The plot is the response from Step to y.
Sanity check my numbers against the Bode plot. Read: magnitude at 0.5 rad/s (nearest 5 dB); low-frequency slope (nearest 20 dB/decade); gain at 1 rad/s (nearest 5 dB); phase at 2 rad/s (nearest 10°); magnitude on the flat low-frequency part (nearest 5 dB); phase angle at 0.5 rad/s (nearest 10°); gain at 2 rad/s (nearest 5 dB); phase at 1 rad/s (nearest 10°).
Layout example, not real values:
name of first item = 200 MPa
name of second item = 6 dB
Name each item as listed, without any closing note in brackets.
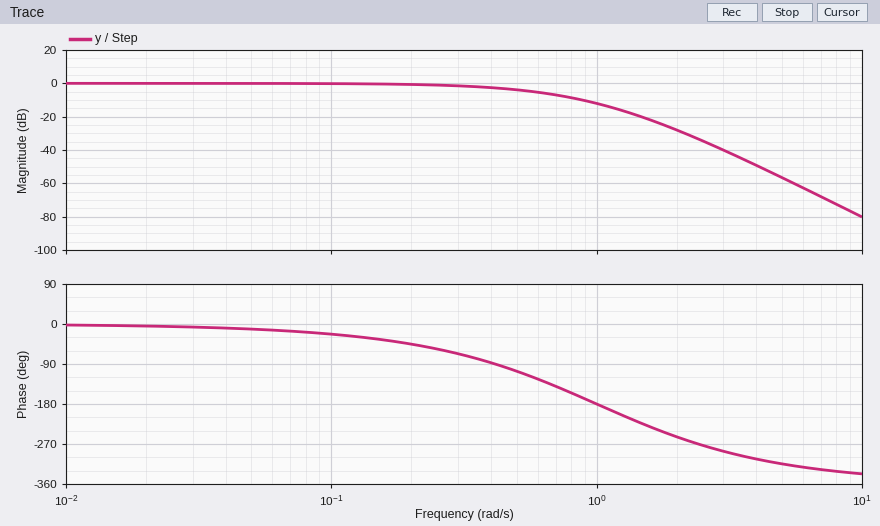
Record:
magnitude at 0.5 rad/s = -5 dB
low-frequency slope = 0 dB/decade
gain at 1 rad/s = -10 dB
phase at 2 rad/s = -250°
magnitude on the flat low-frequency part = 0 dB
phase angle at 0.5 rad/s = -110°
gain at 2 rad/s = -30 dB
phase at 1 rad/s = -180°
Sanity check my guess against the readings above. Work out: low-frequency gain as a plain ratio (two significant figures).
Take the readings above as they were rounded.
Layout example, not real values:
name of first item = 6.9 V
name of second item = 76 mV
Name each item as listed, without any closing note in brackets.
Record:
low-frequency gain as a plain ratio = 1.0
